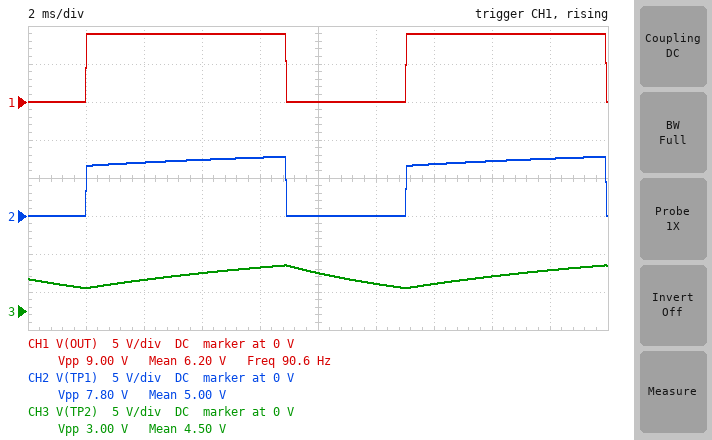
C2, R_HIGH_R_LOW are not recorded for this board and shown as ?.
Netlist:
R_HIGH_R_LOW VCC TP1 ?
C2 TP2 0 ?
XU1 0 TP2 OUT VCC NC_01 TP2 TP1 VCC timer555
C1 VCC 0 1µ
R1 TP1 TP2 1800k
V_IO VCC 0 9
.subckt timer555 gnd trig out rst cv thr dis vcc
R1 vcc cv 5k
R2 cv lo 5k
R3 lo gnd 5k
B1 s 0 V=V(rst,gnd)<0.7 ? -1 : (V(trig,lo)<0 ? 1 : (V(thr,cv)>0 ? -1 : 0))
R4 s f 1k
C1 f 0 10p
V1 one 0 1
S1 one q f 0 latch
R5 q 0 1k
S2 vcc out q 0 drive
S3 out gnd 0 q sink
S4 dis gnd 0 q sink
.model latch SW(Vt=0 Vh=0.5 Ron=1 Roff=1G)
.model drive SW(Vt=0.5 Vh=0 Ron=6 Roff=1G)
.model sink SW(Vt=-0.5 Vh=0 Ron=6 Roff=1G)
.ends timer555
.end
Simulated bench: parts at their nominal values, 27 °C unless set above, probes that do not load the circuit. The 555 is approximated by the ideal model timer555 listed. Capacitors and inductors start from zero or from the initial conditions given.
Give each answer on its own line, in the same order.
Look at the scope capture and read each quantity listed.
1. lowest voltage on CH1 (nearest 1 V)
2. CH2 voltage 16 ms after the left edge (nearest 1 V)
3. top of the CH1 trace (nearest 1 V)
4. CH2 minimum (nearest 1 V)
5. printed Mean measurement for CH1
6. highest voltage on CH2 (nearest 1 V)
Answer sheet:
0 V
7 V
9 V
0 V
6.20 V
8 V
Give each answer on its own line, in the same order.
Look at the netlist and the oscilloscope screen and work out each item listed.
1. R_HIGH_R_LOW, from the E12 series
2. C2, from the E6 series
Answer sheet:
1.2 MΩ
3.3 nF
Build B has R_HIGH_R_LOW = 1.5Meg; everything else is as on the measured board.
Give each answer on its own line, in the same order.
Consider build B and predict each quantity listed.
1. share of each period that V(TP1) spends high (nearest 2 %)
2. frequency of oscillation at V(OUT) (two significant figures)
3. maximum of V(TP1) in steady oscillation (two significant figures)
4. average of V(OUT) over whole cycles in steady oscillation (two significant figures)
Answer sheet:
64 %
86 Hz
7.6 V
5.8 V
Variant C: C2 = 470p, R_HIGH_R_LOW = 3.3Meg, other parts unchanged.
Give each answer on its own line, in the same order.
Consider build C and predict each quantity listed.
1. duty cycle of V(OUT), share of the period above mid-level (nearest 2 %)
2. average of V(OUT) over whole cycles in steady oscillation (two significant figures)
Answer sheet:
74 %
6.7 V
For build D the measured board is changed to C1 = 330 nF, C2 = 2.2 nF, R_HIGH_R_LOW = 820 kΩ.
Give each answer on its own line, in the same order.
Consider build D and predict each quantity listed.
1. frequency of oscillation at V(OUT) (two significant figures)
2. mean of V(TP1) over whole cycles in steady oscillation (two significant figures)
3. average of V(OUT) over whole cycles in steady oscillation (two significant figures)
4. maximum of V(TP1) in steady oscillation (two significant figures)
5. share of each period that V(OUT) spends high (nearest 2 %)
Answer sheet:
150 Hz
4.5 V
5.3 V
8.1 V
60 %
